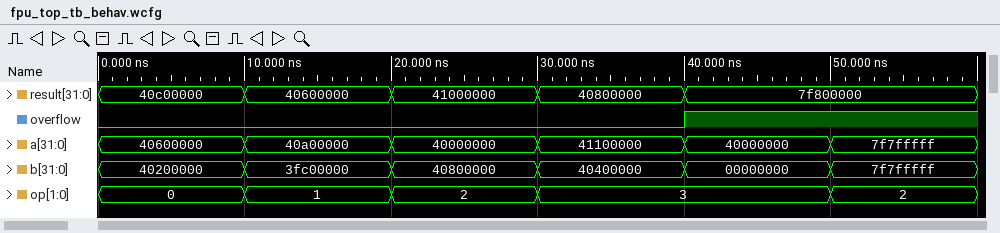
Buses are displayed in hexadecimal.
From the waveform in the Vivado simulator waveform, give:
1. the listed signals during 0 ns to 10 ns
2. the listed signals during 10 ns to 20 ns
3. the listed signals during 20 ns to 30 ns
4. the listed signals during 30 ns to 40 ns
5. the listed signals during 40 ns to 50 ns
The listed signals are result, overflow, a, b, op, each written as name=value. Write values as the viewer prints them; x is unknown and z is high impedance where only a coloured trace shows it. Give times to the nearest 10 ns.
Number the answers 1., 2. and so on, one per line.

1. result=40c00000, overflow=0, a=40600000, b=40200000, op=0
2. result=40600000, overflow=0, a=40a00000, b=3fc00000, op=1
3. result=41000000, overflow=0, a=40000000, b=40800000, op=2
4. result=40800000, overflow=0, a=41100000, b=40400000, op=3
5. result=7f800000, overflow=1, a=40000000, b=00000000, op=3
